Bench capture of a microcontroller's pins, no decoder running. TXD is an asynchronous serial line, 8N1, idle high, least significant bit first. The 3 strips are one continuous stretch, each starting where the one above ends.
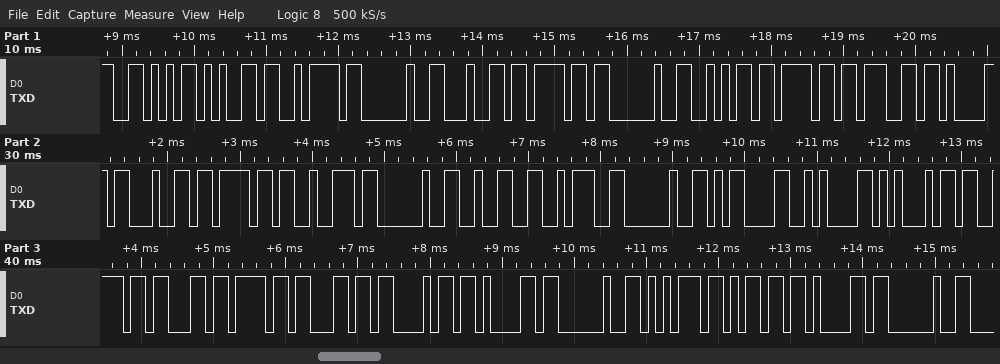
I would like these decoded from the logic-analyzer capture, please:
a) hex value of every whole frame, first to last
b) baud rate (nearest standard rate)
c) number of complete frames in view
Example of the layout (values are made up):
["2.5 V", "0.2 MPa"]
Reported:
["56 65 7A 20 64 6F 20 6A 6F 67 61 64 6F 72 20 32 3A 20 0D 0A 45 73 63 6F 6C 68 61 20 75 6D 61 20", "9600 baud", "32"]
